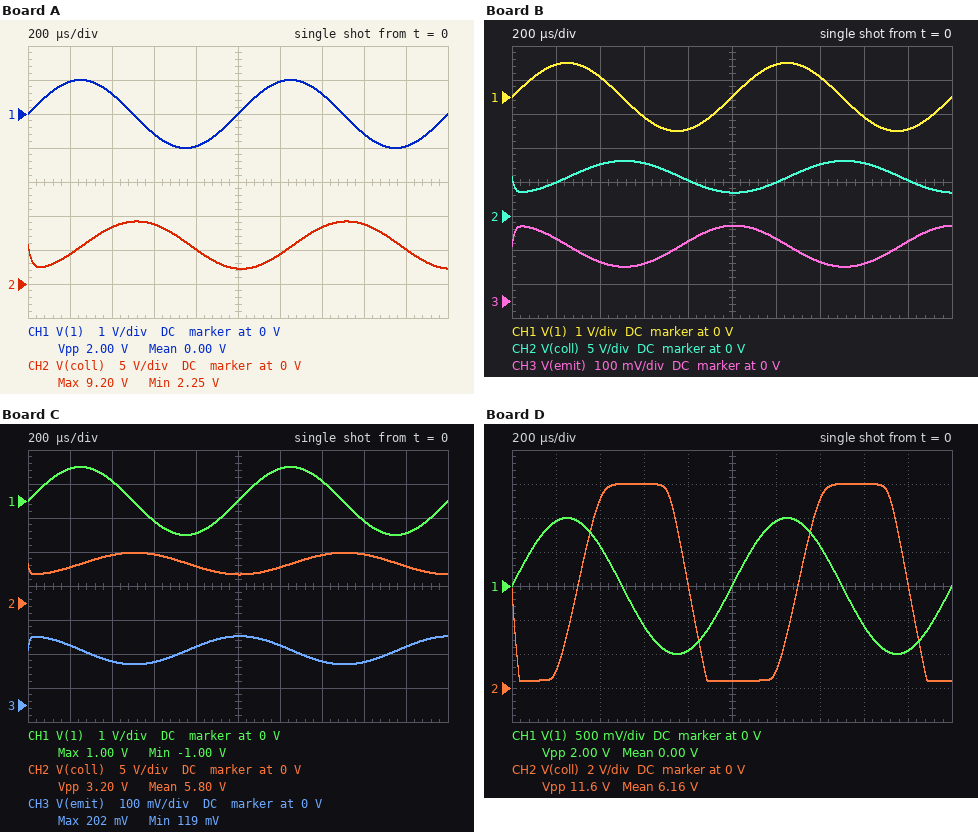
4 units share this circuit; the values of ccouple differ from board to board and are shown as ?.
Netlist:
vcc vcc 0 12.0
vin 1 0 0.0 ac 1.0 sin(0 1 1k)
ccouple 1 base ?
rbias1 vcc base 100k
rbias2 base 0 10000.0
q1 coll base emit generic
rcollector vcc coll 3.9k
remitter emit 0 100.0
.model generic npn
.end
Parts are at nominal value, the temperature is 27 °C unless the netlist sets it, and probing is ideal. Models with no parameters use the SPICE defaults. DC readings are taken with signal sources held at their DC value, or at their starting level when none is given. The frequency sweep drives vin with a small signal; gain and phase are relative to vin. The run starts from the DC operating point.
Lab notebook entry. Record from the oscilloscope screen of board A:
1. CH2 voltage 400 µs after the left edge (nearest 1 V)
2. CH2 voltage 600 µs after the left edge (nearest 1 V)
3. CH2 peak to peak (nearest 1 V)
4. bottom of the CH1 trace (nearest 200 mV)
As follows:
8 V
9 V
7 V
-1.0 V
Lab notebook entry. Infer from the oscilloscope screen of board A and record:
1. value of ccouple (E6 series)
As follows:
3.3 nF
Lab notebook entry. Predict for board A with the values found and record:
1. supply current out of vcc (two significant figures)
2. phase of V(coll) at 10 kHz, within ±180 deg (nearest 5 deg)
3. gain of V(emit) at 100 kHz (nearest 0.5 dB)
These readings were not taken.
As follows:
1.7 mA
-135 deg
-1.5 dB
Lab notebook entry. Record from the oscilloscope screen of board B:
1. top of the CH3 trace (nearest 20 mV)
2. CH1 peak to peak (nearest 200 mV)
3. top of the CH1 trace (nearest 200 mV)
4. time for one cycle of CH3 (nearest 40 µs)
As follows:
220 mV
2.0 V
1.0 V
1.00 ms
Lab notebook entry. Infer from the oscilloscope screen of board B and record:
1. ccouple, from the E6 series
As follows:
2.2 nF
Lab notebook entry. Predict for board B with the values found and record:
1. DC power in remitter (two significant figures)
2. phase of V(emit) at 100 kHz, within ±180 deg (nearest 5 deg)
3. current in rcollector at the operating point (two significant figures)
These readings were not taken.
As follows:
260 µW
10 deg
1.6 mA
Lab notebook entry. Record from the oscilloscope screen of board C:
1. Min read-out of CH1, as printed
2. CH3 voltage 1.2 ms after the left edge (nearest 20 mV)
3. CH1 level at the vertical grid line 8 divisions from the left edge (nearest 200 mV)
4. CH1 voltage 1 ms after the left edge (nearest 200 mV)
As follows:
-1.00 V
180 mV
-600 mV
0 V
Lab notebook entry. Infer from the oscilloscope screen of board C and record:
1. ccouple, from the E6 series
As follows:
1.5 nF
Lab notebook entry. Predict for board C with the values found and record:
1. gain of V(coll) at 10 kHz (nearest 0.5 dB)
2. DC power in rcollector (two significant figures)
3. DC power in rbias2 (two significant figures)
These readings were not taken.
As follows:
23.0 dB
9.8 mW
90 µW
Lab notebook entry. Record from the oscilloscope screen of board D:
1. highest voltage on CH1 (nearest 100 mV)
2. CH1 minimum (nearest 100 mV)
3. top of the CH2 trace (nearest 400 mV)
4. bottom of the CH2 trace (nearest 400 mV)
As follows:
1.0 V
-1.0 V
12.0 V
400 mV
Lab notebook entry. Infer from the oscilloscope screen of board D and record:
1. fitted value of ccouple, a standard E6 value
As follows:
10 nF
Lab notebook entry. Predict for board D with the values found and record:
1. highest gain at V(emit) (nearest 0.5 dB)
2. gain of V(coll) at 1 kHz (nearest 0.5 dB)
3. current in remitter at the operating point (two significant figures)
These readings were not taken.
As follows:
-1.5 dB
20.0 dB
1.6 mA
